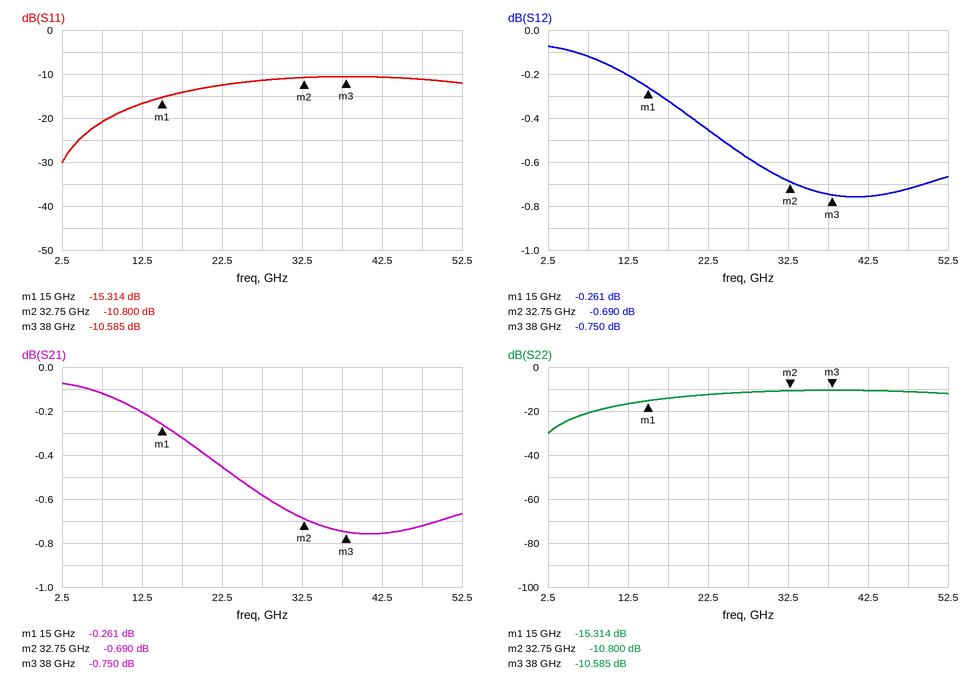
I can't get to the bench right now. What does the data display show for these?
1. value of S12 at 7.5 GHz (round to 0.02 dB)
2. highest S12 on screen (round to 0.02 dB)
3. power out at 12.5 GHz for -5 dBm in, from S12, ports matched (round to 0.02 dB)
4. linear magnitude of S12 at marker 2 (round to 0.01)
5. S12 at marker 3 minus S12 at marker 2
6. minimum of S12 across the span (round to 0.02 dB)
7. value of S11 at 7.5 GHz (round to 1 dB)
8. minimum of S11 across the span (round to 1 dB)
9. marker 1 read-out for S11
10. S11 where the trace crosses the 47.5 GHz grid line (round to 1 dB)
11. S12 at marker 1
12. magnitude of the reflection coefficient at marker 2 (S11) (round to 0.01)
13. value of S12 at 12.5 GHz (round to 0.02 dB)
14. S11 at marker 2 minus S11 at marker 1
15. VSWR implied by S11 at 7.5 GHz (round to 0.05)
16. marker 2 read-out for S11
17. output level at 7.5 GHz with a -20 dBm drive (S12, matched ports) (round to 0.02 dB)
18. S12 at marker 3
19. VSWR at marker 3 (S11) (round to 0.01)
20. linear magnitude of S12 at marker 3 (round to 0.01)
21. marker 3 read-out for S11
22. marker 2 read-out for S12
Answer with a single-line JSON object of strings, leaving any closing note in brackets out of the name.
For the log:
{"value of S12 at 7.5 GHz": "-0.12 dB", "highest S12 on screen": "-0.08 dB", "power out at 12.5 GHz for -5 dBm in, from S12, ports matched": "-5.20 dBm", "linear magnitude of S12 at marker 2": "0.92", "S12 at marker 3 minus S12 at marker 2": "-0.060 dB", "minimum of S12 across the span": "-0.76 dB", "value of S11 at 7.5 GHz": "-21 dB", "minimum of S11 across the span": "-30 dB", "marker 1 read-out for S11": "-15.314 dB", "S11 where the trace crosses the 47.5 GHz grid line": "-11 dB", "S12 at marker 1": "-0.261 dB", "magnitude of the reflection coefficient at marker 2 (S11)": "0.29", "value of S12 at 12.5 GHz": "-0.20 dB", "S11 at marker 2 minus S11 at marker 1": "4.514 dB", "VSWR implied by S11 at 7.5 GHz": "1.20", "marker 2 read-out for S11": "-10.800 dB", "output level at 7.5 GHz with a -20 dBm drive (S12, matched ports)": "-20.12 dBm", "S12 at marker 3": "-0.750 dB", "VSWR at marker 3 (S11)": "1.84", "linear magnitude of S12 at marker 3": "0.92", "marker 3 read-out for S11": "-10.585 dB", "marker 2 read-out for S12": "-0.690 dB"}
